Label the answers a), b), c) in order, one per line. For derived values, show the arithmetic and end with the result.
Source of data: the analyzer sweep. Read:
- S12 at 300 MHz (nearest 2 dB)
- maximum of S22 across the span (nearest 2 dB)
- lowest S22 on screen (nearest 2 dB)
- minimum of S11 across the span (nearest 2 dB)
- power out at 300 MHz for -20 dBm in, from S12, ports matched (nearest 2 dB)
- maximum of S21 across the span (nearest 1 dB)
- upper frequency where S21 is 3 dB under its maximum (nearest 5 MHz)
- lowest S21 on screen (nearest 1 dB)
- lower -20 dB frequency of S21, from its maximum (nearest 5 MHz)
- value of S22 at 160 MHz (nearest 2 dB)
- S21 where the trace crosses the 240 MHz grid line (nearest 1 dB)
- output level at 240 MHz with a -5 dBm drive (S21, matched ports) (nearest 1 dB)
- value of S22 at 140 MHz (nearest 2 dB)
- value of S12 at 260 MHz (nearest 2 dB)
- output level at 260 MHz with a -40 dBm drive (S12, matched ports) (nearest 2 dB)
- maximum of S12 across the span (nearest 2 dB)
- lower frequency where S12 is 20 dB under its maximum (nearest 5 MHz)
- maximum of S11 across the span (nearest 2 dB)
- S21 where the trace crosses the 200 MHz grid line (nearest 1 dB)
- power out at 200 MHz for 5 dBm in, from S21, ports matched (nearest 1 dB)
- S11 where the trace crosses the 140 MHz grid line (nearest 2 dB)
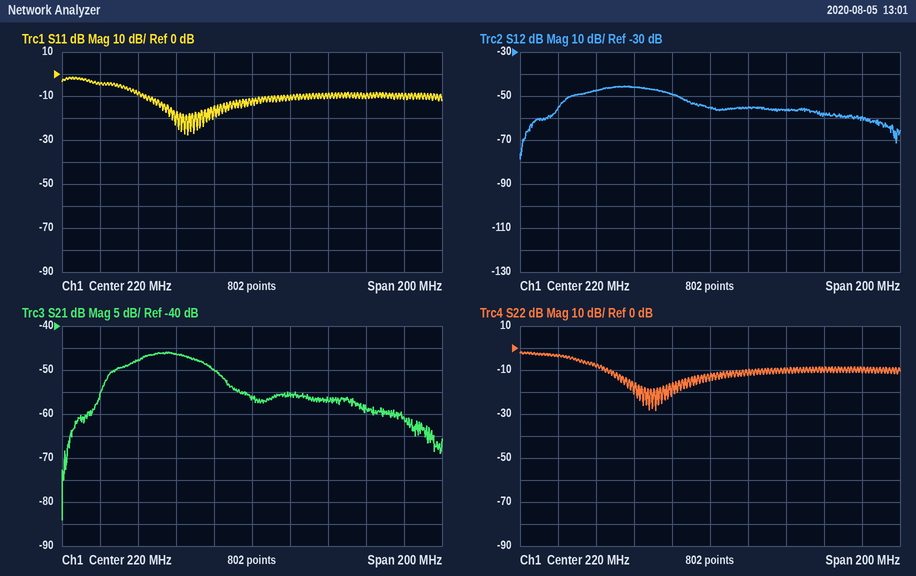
a) -60 dB
b) -2 dB
c) -28 dB
d) -28 dB
e) -20 dBm + (-60 dB) = -80 dBm
f) -46 dB
g) 195 MHz
h) -84 dB
i) 125 MHz
j) -8 dB
k) -55 dB
l) -5 dBm + (-55 dB) = -60 dBm
m) -4 dB
n) -56 dB
o) -40 dBm + (-56 dB) = -96 dBm
p) -46 dB
q) 125 MHz
r) -2 dB
s) -50 dB
t) 5 dBm + (-50 dB) = -45 dBm
u) -4 dB
